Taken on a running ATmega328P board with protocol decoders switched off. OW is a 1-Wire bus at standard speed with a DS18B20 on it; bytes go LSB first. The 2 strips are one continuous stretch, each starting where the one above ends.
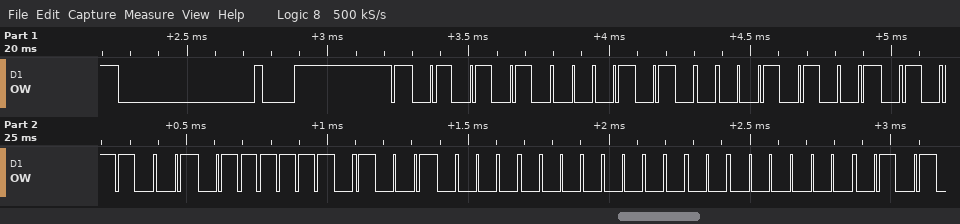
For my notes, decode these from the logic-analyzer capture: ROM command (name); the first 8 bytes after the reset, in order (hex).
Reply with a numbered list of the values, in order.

1. Match ROM
2. 55 28 94 9A 7E 09 00 00
